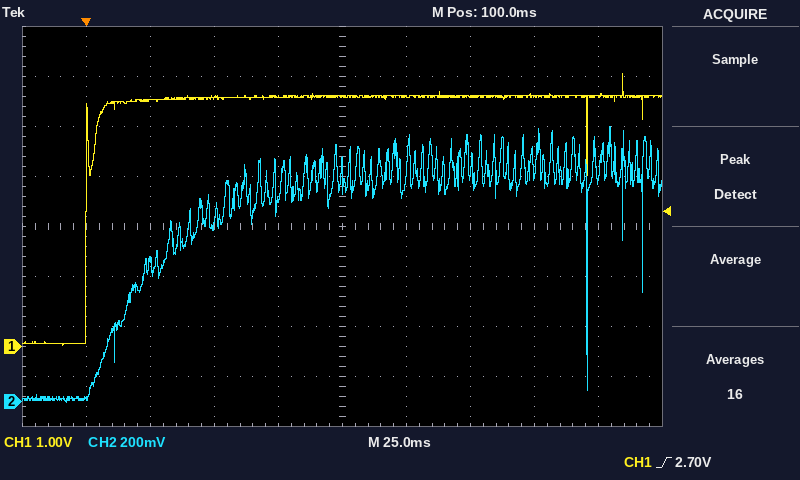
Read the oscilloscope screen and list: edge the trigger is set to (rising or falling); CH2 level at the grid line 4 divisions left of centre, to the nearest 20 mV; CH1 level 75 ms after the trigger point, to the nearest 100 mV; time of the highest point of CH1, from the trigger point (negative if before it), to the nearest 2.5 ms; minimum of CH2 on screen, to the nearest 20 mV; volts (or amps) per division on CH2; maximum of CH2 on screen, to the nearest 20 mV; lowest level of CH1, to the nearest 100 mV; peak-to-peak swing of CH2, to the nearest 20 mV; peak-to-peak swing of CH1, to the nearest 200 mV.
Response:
rising
20 mV
5.0 V
+210.0 ms
0 mV
200 mV
1.10 V
0.0 V
1.10 V
5.4 V
